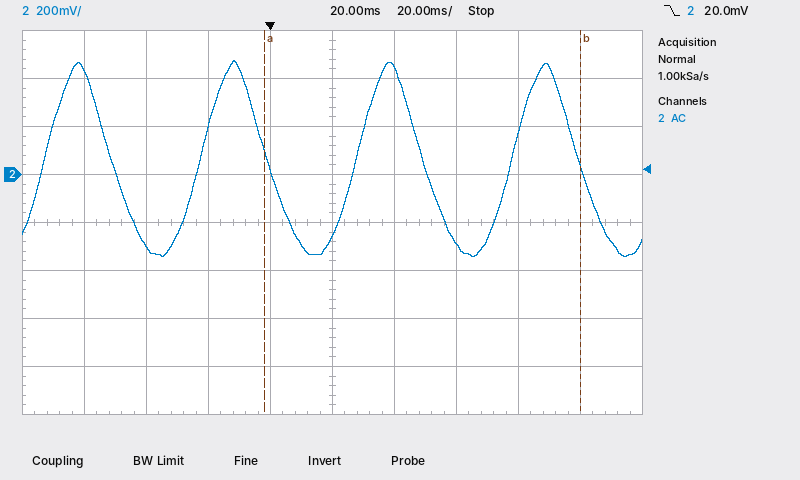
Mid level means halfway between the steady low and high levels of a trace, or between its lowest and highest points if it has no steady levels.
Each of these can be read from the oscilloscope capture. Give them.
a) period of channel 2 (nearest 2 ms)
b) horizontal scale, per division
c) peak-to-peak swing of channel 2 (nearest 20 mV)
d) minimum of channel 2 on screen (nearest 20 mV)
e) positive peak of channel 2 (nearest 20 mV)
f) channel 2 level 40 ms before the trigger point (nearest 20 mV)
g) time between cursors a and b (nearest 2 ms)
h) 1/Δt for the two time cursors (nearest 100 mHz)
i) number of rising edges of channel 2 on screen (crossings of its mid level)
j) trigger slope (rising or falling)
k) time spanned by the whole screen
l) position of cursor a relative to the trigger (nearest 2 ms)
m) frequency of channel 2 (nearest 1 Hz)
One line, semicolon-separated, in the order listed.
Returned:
50 ms; 20 ms; 820 mV; -340 mV; 480 mV; -300 mV; 102 ms; 9.8 Hz; 4; falling; 200 ms; -2 ms; 20 Hz
